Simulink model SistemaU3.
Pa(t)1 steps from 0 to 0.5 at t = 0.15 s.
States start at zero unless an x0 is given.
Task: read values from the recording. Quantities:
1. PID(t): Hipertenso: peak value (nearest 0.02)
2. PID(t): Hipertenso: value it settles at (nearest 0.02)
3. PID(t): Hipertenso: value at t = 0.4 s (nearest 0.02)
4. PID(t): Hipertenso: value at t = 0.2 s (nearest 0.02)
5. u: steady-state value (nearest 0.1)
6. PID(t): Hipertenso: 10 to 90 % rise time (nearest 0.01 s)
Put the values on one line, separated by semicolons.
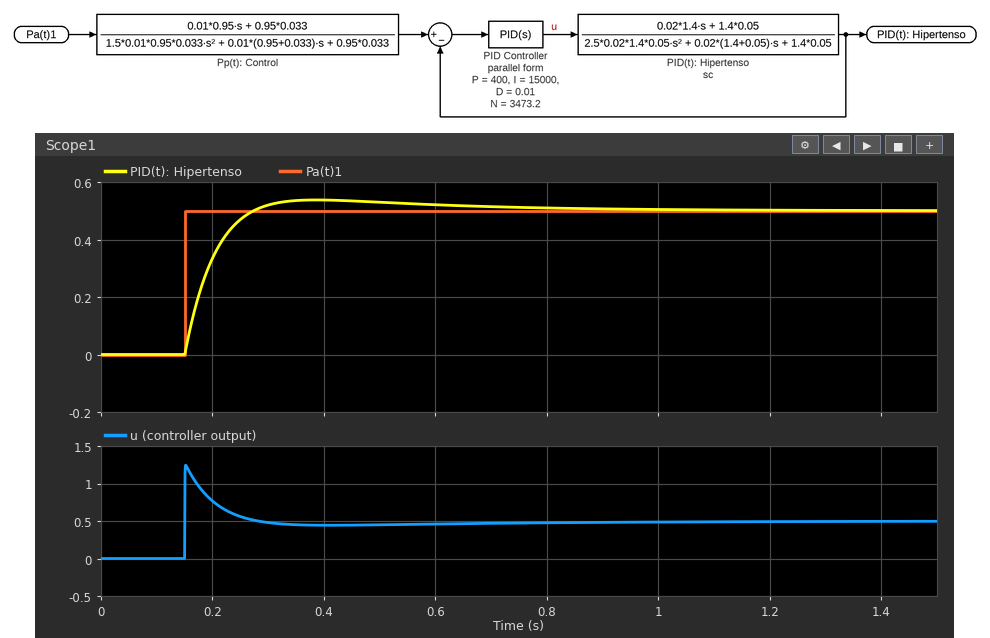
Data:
0.54; 0.50; 0.54; 0.34; 0.5; 0.08 s
